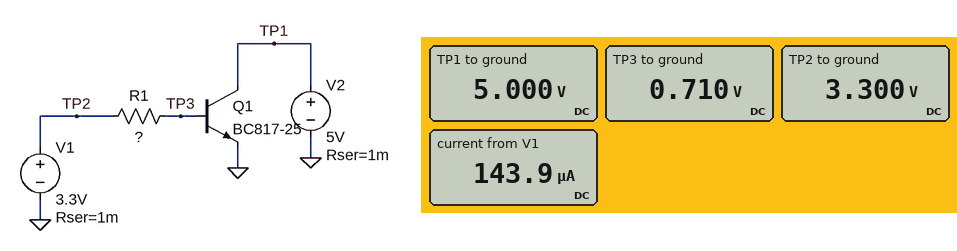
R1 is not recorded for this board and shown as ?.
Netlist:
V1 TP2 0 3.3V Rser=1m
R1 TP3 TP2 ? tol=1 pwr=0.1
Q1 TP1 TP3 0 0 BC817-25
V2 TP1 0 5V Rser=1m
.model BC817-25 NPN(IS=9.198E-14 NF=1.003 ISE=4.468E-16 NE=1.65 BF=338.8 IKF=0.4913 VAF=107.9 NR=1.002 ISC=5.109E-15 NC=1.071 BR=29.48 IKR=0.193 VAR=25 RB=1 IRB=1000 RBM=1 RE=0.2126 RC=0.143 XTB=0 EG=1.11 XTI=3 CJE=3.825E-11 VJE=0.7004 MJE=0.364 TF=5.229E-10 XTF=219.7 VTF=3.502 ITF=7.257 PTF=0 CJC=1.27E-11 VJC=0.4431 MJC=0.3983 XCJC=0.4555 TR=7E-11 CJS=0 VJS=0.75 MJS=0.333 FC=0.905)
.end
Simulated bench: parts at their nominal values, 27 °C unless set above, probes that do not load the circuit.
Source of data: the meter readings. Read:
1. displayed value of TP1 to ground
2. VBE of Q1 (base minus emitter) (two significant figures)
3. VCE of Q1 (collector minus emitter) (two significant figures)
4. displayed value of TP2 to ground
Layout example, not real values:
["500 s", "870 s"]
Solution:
["5.000 V", "710 mV", "5.0 V", "3.300 V"]
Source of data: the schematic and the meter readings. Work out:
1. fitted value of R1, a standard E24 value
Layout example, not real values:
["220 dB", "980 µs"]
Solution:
["18 kΩ"]
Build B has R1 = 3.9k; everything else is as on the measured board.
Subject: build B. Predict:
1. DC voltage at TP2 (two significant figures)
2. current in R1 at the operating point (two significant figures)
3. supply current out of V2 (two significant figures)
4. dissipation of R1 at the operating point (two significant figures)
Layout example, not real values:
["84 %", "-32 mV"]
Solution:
["3.3 V", "650 µA", "170 mA", "1.6 mW"]
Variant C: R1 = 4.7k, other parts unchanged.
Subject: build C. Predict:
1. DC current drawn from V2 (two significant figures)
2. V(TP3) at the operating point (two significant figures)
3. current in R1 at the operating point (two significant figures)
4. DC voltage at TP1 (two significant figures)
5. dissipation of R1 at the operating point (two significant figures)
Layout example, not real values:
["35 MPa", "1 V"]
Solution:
["140 mA", "770 mV", "540 µA", "5.0 V", "1.4 mW"]
